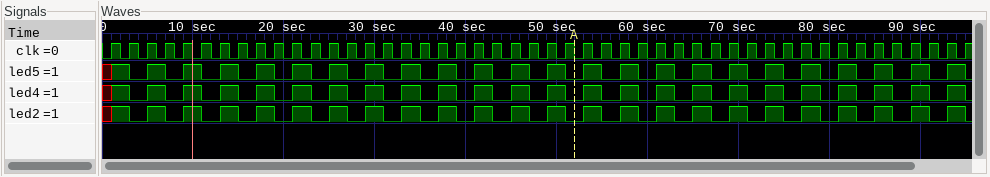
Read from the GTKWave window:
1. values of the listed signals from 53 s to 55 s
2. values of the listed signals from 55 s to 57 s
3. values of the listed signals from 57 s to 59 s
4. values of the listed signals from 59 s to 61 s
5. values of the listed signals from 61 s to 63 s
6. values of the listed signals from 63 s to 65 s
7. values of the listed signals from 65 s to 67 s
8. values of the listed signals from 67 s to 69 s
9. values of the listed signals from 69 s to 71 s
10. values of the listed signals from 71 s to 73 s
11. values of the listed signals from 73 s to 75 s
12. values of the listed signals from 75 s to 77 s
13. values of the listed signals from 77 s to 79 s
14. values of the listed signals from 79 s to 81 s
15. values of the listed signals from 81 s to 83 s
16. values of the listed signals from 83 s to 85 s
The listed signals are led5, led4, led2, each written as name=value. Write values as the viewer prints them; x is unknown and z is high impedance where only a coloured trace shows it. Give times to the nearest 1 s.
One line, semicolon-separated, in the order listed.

led5=1, led4=1, led2=1; led5=0, led4=0, led2=0; led5=1, led4=1, led2=1; led5=0, led4=0, led2=0; led5=1, led4=1, led2=1; led5=0, led4=0, led2=0; led5=1, led4=1, led2=1; led5=0, led4=0, led2=0; led5=1, led4=1, led2=1; led5=0, led4=0, led2=0; led5=1, led4=1, led2=1; led5=0, led4=0, led2=0; led5=1, led4=1, led2=1; led5=0, led4=0, led2=0; led5=1, led4=1, led2=1; led5=0, led4=0, led2=0
